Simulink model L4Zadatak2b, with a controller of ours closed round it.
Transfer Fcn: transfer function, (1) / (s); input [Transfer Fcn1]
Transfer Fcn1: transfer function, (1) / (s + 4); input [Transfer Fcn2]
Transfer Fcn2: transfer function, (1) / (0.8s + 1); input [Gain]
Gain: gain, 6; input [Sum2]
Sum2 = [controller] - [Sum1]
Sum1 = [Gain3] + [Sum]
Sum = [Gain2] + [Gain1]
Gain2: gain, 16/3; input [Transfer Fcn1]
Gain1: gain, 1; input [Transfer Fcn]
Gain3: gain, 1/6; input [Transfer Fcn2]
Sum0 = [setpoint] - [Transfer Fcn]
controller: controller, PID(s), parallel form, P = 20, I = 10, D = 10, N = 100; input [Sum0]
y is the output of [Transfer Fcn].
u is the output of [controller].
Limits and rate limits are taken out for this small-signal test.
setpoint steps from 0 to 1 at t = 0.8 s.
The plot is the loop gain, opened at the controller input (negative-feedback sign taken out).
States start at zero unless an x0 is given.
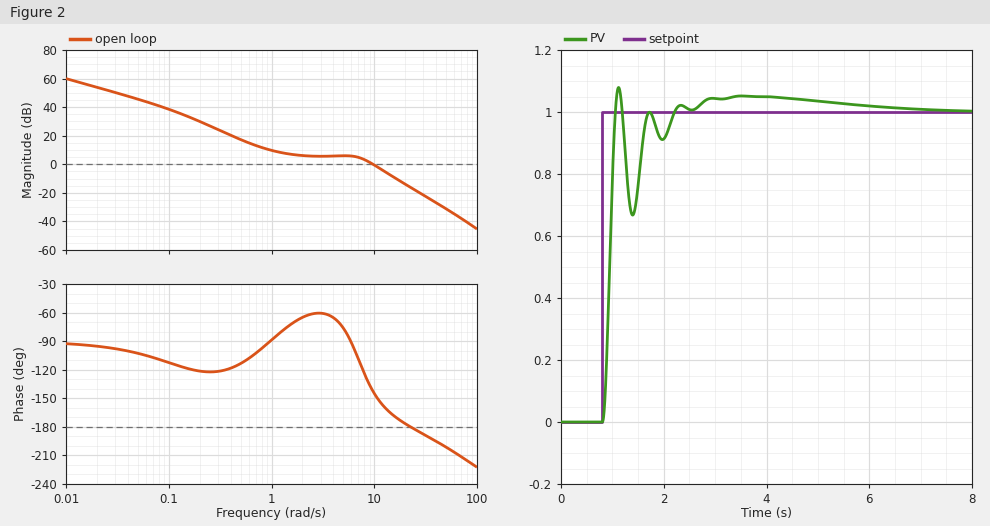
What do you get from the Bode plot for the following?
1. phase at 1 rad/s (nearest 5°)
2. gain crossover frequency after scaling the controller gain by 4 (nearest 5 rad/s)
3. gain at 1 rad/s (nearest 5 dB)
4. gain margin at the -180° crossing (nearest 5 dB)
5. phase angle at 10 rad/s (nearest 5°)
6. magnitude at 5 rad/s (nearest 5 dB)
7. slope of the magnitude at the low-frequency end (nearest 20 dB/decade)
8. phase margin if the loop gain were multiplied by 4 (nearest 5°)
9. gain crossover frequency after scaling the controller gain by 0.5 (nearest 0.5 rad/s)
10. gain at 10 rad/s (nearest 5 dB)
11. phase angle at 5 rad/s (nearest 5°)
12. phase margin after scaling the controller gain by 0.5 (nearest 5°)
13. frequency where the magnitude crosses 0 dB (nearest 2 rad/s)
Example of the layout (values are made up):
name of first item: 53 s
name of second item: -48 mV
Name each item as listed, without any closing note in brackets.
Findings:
phase at 1 rad/s: -90°
gain crossover frequency after scaling the controller gain by 4: 20 rad/s
gain at 1 rad/s: 10 dB
gain margin at the -180° crossing: 15 dB
phase angle at 10 rad/s: -145°
magnitude at 5 rad/s: 5 dB
slope of the magnitude at the low-frequency end: -20 dB/decade
phase margin if the loop gain were multiplied by 4: 5°
gain crossover frequency after scaling the controller gain by 0.5: 2.0 rad/s
gain at 10 rad/s: 0 dB
phase angle at 5 rad/s: -75°
phase margin after scaling the controller gain by 0.5: 115°
frequency where the magnitude crosses 0 dB: 10 rad/s
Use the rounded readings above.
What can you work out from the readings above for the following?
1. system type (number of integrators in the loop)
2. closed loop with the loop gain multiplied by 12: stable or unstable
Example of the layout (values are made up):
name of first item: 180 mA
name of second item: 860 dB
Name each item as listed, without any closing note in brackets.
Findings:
system type: 1
closed loop with the loop gain multiplied by 12: stable or unstable: unstable
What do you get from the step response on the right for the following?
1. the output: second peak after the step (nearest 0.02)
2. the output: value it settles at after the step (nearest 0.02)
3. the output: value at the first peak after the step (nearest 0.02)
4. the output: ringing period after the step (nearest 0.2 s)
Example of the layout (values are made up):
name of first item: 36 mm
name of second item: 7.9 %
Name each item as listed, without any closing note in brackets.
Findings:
the output: second peak after the step: 1.00
the output: value it settles at after the step: 1.00
the output: value at the first peak after the step: 1.08
the output: ringing period after the step: 0.6 s
